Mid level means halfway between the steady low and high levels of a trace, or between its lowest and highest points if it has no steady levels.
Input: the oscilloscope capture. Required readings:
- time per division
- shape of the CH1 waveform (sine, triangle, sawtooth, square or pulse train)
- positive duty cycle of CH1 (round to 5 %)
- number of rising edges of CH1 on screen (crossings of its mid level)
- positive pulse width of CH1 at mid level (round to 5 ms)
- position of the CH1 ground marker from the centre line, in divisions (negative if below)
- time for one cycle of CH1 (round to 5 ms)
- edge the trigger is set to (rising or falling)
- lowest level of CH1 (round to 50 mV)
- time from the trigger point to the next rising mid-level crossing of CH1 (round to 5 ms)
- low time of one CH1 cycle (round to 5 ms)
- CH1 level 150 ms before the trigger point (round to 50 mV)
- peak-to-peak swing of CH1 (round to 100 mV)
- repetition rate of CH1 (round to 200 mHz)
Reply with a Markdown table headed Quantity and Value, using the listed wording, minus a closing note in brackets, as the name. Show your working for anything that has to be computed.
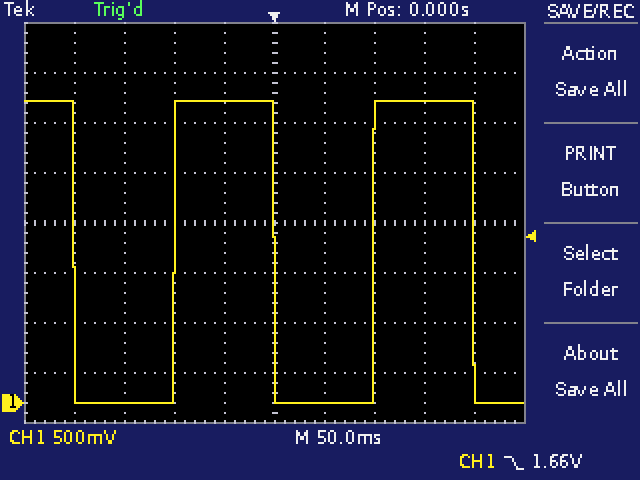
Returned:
| Quantity | Value |
|---|---|
| time per division | 50 ms |
| shape of the CH1 waveform | square |
| positive duty cycle of CH1 | 100 ms / 200 ms ≈ 50 % |
| number of rising edges of CH1 on screen | 2 |
| positive pulse width of CH1 at mid level | 100 ms |
| position of the CH1 ground marker from the centre line, in divisions | -3.6 div |
| time for one cycle of CH1 | 200 ms |
| edge the trigger is set to | falling |
| lowest level of CH1 | 0 mV |
| time from the trigger point to the next rising mid-level crossing of CH1 | 100 ms |
| low time of one CH1 cycle | 100 ms |
| CH1 level 150 ms before the trigger point | 0 mV |
| peak-to-peak swing of CH1 | 3.00 V |
| repetition rate of CH1 | 1 / 200 ms ≈ 5.0 Hz |
